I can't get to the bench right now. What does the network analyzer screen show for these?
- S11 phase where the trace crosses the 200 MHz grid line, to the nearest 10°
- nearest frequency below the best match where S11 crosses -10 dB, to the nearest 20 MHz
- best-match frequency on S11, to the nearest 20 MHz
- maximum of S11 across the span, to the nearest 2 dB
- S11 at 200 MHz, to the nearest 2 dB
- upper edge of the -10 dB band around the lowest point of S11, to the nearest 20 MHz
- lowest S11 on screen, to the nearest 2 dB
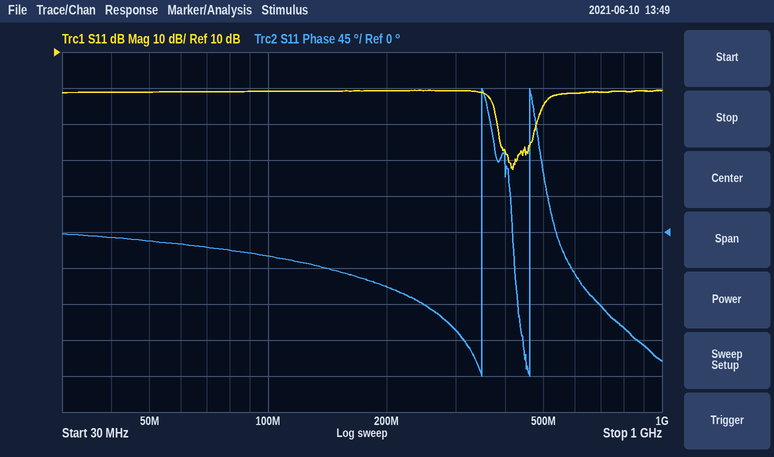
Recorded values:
-70°
380 MHz
420 MHz
0 dB
0 dB
480 MHz
-22 dB
